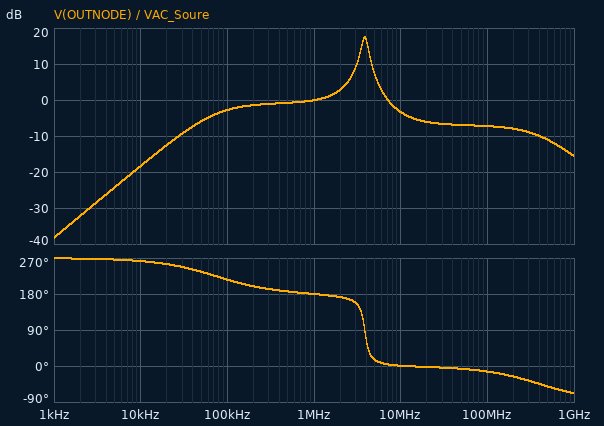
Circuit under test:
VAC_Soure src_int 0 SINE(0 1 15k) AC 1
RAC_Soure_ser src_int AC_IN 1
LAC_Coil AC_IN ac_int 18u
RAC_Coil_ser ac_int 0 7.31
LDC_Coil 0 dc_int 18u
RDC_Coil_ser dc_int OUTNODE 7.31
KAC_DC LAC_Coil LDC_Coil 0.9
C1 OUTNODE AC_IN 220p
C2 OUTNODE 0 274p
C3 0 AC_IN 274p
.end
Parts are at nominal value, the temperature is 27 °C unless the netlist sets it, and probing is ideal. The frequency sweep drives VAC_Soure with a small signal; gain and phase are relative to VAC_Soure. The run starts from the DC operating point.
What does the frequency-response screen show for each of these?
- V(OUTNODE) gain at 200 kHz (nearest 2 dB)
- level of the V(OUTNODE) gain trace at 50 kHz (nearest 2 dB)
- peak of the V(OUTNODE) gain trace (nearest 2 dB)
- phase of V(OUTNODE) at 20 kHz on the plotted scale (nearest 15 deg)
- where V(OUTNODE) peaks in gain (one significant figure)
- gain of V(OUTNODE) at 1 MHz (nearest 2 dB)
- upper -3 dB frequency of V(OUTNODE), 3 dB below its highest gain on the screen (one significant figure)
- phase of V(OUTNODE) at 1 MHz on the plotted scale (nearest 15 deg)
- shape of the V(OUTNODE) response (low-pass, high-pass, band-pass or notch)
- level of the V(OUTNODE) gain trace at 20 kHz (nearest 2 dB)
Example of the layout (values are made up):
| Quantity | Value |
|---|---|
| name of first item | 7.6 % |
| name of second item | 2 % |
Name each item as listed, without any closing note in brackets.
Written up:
| Quantity | Value |
|---|---|
| V(OUTNODE) gain at 200 kHz | -2 dB |
| level of the V(OUTNODE) gain trace at 50 kHz | -6 dB |
| peak of the V(OUTNODE) gain trace | 18 dB |
| phase of V(OUTNODE) at 20 kHz on the plotted scale | 255 deg |
| where V(OUTNODE) peaks in gain | 4 MHz |
| gain of V(OUTNODE) at 1 MHz | 0 dB |
| upper -3 dB frequency of V(OUTNODE), 3 dB below its highest gain on the screen | 4 MHz |
| phase of V(OUTNODE) at 1 MHz on the plotted scale | 180 deg |
| shape of the V(OUTNODE) response | band-pass |
| level of the V(OUTNODE) gain trace at 20 kHz | -12 dB |
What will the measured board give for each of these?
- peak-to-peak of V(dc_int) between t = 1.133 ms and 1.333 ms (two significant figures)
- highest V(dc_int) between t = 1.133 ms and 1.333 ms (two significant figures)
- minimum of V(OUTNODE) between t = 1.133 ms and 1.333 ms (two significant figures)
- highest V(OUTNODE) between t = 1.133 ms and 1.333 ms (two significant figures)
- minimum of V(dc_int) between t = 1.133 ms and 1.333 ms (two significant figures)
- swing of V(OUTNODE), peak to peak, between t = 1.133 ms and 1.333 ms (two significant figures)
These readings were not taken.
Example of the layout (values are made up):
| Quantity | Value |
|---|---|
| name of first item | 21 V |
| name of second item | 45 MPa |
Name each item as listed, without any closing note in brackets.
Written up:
| Quantity | Value |
|---|---|
| peak-to-peak of V(dc_int) between t = 1.133 ms and 1.333 ms | 360 mV |
| highest V(dc_int) between t = 1.133 ms and 1.333 ms | 180 mV |
| minimum of V(OUTNODE) between t = 1.133 ms and 1.333 ms | -180 mV |
| highest V(OUTNODE) between t = 1.133 ms and 1.333 ms | 180 mV |
| minimum of V(dc_int) between t = 1.133 ms and 1.333 ms | -180 mV |
| swing of V(OUTNODE), peak to peak, between t = 1.133 ms and 1.333 ms | 360 mV |
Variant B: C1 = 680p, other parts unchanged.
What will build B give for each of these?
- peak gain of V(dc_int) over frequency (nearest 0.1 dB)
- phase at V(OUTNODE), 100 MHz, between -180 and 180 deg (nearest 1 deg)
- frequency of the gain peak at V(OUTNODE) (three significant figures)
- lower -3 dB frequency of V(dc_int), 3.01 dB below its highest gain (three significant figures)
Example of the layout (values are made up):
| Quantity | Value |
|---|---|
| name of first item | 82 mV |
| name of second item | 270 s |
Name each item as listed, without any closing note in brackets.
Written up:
| Quantity | Value |
|---|---|
| peak gain of V(dc_int) over frequency | 15.7 dB |
| phase at V(OUTNODE), 100 MHz, between -180 and 180 deg | -16 deg |
| frequency of the gain peak at V(OUTNODE) | 2.78 MHz |
| lower -3 dB frequency of V(dc_int), 3.01 dB below its highest gain | 2.42 MHz |
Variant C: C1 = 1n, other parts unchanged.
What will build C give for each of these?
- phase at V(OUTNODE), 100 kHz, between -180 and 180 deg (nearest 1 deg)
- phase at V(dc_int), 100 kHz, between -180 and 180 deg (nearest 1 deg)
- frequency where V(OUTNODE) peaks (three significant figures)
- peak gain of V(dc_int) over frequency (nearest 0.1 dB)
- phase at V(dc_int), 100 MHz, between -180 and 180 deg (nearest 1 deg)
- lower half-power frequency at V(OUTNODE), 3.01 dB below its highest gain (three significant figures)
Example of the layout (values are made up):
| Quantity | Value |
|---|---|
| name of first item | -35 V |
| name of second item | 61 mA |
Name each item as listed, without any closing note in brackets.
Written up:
| Quantity | Value |
|---|---|
| phase at V(OUTNODE), 100 kHz, between -180 and 180 deg | -145 deg |
| phase at V(dc_int), 100 kHz, between -180 and 180 deg | -144 deg |
| frequency where V(OUTNODE) peaks | 2.40 MHz |
| peak gain of V(dc_int) over frequency | 14.7 dB |
| phase at V(dc_int), 100 MHz, between -180 and 180 deg | -17 deg |
| lower half-power frequency at V(OUTNODE), 3.01 dB below its highest gain | 2.05 MHz |
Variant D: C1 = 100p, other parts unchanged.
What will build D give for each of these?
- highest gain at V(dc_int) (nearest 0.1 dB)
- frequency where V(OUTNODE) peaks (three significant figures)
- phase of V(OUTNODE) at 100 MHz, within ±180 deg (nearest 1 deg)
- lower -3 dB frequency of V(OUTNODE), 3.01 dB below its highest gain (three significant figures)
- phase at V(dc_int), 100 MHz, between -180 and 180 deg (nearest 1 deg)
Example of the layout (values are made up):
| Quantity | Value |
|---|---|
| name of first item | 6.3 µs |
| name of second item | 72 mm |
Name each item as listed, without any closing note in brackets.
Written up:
| Quantity | Value |
|---|---|
| highest gain at V(dc_int) | 17.7 dB |
| frequency where V(OUTNODE) peaks | 4.43 MHz |
| phase of V(OUTNODE) at 100 MHz, within ±180 deg | -12 deg |
| lower -3 dB frequency of V(OUTNODE), 3.01 dB below its highest gain | 4.09 MHz |
| phase at V(dc_int), 100 MHz, between -180 and 180 deg | -11 deg |
